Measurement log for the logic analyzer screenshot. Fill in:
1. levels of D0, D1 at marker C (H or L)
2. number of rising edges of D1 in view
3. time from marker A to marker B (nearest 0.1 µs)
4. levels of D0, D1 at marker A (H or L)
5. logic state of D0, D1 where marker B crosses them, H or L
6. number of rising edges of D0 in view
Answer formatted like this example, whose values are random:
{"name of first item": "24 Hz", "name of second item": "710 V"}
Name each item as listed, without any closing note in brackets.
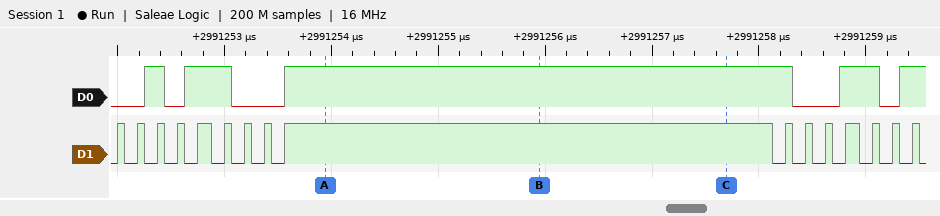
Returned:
{"levels of D0, D1 at marker C": "D0=H, D1=H", "number of rising edges of D1 in view": "16", "time from marker A to marker B": "2 µs", "levels of D0, D1 at marker A": "D0=H, D1=H", "logic state of D0, D1 where marker B crosses them, H or L": "D0=H, D1=H", "number of rising edges of D0 in view": "5"}
